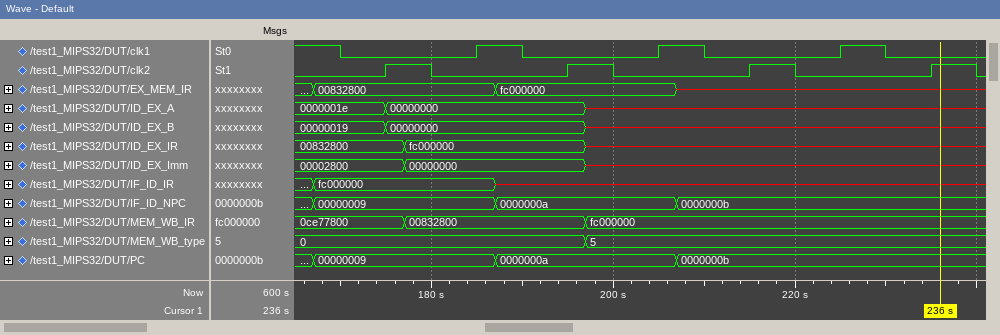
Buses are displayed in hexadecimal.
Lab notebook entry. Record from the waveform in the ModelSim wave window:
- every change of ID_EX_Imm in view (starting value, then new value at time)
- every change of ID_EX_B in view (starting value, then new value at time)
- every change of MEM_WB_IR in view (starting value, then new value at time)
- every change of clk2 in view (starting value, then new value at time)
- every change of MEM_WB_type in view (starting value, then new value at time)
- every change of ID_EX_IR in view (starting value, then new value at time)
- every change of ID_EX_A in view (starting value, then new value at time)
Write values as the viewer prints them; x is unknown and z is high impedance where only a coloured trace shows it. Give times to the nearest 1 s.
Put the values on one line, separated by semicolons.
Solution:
00002800, 00000000 at 177 s, x at 197 s; 00000019, 00000000 at 175 s, x at 197 s; 0ce77800, 00832800 at 177 s, fc000000 at 197 s; 0, 1 at 175 s, 0 at 180 s, 1 at 195 s, 0 at 200 s, 1 at 215 s, 0 at 220 s, 1 at 235 s, 0 at 240 s; 0, 5 at 197 s; 00832800, fc000000 at 177 s, x at 197 s; 0000001e, 00000000 at 175 s, x at 197 s
